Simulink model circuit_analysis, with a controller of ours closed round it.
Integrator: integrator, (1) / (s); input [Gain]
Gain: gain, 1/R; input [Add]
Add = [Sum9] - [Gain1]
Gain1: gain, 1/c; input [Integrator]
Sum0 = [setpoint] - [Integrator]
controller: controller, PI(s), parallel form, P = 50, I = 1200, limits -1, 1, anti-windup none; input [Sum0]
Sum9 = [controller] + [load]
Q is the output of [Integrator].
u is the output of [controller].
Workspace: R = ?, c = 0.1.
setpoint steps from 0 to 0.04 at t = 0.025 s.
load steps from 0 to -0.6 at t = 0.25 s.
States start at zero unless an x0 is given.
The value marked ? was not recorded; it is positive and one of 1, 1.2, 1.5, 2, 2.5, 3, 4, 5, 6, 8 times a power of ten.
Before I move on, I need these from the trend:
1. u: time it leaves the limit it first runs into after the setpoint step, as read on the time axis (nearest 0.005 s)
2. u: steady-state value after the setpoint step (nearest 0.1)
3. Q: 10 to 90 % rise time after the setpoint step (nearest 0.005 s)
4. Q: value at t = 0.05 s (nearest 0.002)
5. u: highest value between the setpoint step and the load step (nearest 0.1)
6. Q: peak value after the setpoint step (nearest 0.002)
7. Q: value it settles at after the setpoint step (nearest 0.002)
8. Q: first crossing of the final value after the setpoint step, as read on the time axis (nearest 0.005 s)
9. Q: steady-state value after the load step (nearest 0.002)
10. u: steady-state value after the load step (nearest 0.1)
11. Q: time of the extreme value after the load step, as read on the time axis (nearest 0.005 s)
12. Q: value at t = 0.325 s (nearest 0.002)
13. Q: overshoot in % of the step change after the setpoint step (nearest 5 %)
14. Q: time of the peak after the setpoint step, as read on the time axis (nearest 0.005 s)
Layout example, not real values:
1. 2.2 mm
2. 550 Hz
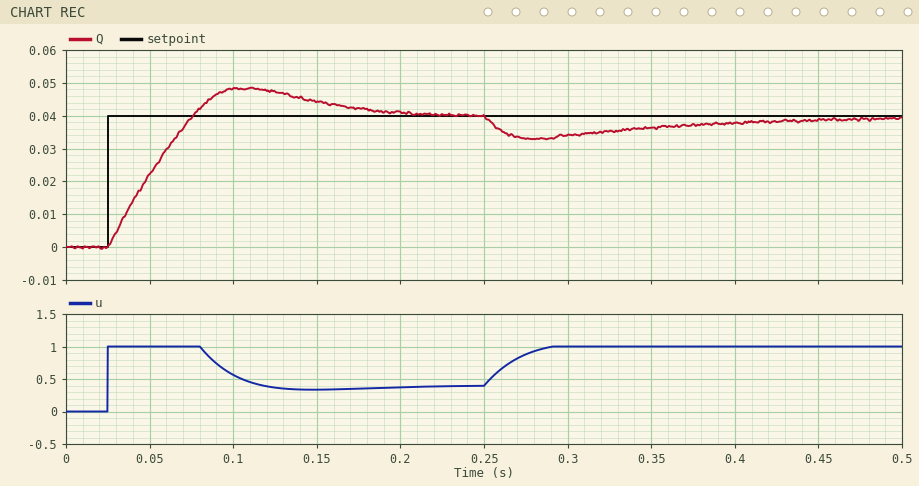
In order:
1. 0.080 s
2. 0.4
3. 0.040 s
4. 0.022
5. 1.0
6. 0.048
7. 0.040
8. 0.075 s
9. 0.040
10. 1.0
11. 0.280 s
12. 0.036
13. 20 %
14. 0.105 s
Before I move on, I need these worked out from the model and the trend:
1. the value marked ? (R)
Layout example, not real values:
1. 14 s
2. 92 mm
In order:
1. 1
